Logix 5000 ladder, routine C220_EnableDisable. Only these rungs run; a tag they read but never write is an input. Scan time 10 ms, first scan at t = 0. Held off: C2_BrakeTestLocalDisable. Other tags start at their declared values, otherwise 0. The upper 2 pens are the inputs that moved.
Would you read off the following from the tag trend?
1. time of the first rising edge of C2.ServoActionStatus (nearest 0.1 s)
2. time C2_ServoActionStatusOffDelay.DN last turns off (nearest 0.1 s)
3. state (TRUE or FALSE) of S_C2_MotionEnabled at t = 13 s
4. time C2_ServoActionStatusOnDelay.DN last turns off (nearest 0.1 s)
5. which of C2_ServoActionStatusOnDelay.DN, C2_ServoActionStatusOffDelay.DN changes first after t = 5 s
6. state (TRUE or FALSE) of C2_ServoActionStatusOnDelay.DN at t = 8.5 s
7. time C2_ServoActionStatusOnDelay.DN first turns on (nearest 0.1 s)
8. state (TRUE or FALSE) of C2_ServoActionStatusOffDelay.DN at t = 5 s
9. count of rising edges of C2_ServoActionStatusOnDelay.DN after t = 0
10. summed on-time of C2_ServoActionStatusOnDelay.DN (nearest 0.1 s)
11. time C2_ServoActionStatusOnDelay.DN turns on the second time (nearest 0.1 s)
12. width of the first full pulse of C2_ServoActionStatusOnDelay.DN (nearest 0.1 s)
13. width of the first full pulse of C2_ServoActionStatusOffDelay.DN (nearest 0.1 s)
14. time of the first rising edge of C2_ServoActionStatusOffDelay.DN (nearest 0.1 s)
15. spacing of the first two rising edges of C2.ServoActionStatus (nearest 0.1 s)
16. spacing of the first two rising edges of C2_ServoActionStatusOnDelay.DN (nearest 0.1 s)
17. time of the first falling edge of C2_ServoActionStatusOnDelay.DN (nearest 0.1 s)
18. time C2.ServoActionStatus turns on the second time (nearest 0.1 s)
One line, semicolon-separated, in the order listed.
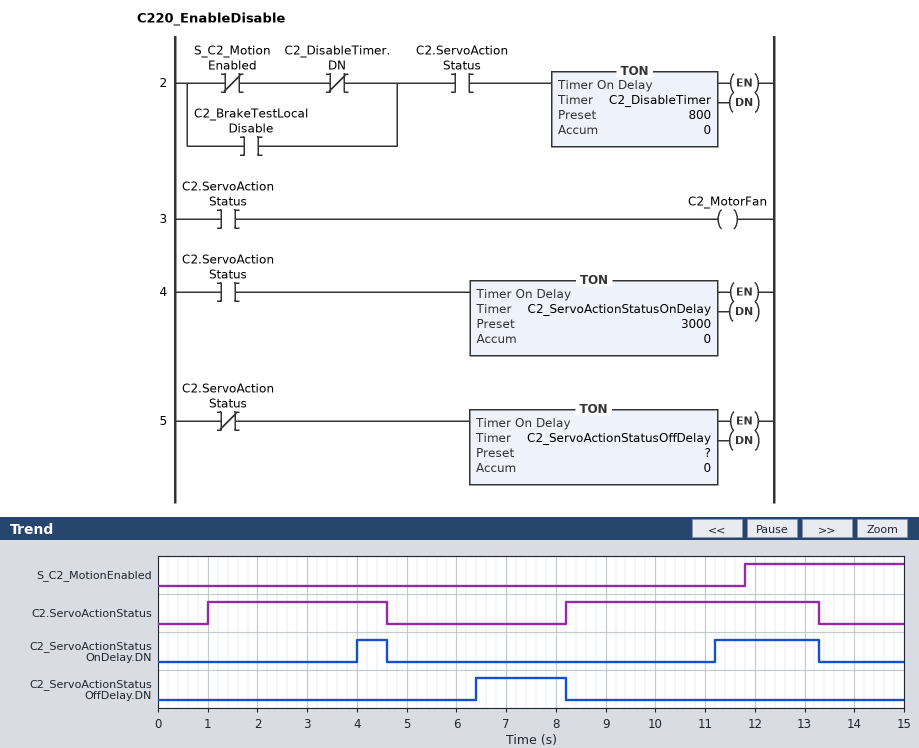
1.0 s; 8.2 s; TRUE; 13.3 s; C2_ServoActionStatusOffDelay.DN; FALSE; 4.0 s; FALSE; 2; 2.7 s; 11.2 s; 0.6 s; 1.8 s; 6.4 s; 7.2 s; 7.2 s; 4.6 s; 8.2 s
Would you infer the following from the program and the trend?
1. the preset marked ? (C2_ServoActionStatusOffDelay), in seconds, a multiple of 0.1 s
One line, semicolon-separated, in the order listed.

1.8 s
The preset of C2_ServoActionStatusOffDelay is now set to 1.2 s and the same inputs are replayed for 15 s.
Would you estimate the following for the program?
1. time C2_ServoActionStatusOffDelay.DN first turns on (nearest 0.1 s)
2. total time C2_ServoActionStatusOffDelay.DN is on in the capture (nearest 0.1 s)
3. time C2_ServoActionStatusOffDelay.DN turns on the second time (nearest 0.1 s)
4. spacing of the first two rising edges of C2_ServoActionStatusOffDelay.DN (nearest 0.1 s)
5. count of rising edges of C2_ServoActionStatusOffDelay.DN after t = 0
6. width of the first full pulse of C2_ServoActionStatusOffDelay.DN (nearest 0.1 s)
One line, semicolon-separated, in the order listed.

5.8 s; 2.9 s; 14.5 s; 8.7 s; 2; 2.4 s
